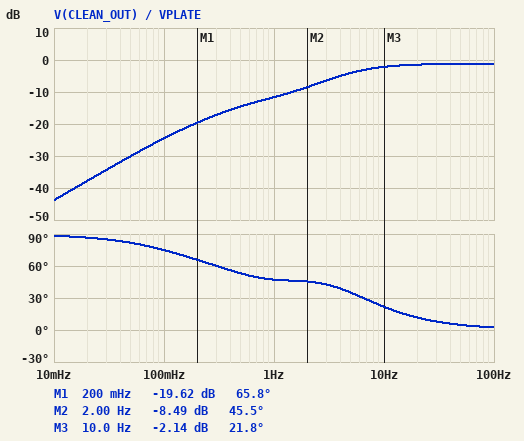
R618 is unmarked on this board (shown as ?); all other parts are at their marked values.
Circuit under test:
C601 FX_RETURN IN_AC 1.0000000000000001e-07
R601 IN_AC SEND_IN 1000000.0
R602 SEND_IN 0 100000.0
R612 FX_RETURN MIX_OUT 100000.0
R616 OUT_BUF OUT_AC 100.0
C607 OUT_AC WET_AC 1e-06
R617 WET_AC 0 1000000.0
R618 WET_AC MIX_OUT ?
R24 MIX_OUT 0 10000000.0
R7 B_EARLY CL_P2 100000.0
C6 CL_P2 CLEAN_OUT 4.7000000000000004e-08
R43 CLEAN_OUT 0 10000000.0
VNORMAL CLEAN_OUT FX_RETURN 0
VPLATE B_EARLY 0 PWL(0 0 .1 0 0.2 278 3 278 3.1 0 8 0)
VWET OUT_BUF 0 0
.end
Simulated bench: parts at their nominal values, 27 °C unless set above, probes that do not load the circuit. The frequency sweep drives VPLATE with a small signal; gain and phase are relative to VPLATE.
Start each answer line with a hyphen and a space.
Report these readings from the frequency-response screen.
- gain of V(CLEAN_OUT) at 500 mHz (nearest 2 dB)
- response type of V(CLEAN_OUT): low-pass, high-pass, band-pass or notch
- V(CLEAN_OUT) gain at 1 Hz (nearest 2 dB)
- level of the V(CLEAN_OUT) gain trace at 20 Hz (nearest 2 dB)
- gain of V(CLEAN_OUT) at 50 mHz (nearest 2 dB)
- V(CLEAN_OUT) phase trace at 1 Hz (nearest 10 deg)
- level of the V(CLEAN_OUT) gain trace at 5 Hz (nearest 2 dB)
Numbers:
- -14 dB
- high-pass
- -12 dB
- -2 dB
- -30 dB
- 50 deg
- -4 dB
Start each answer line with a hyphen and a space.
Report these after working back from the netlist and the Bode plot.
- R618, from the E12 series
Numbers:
- 2.7 MΩ
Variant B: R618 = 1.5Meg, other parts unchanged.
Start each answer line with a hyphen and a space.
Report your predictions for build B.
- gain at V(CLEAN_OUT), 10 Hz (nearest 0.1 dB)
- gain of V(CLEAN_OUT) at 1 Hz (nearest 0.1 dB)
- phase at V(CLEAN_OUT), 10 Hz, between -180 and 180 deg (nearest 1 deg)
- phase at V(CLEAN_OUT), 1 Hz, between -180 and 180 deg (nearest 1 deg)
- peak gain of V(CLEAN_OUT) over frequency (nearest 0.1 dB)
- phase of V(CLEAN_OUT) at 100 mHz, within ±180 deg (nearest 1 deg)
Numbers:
- -2.5 dB
- -13.2 dB
- 25 deg
- 53 deg
- -1.4 dB
- 74 deg
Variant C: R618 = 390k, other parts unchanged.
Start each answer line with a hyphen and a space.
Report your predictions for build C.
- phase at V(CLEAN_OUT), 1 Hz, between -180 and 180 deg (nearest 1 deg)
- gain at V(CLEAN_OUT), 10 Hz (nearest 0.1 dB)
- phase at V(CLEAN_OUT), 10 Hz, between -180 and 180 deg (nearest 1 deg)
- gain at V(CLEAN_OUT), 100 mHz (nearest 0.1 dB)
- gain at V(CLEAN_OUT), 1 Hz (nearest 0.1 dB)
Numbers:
- 59 deg
- -4.7 dB
- 37 deg
- -30.5 dB
- -18.8 dB
